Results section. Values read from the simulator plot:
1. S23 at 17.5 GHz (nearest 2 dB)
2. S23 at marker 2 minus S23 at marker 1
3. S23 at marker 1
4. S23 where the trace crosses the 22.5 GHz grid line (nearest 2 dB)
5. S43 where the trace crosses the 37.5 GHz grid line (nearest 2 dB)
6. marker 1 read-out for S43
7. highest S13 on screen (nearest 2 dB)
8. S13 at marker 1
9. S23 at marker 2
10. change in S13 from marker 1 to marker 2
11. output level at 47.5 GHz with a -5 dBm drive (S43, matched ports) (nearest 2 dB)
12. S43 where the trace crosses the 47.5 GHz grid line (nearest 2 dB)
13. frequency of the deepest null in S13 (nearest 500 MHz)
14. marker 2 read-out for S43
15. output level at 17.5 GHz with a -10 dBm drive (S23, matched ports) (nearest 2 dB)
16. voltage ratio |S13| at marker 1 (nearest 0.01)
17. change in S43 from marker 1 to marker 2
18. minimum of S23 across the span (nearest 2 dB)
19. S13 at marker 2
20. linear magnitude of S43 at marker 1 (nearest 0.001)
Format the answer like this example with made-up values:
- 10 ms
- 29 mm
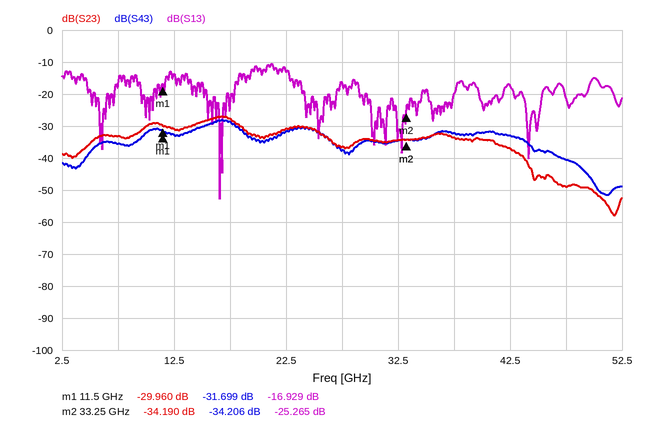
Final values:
- -28 dB
- -4.230 dB
- -29.960 dB
- -30 dB
- -32 dB
- -31.699 dB
- -10 dB
- -16.929 dB
- -34.190 dB
- -8.336 dB
- -46 dBm
- -40 dB
- 16.5 GHz
- -34.206 dB
- -38 dBm
- 0.14
- -2.507 dB
- -58 dB
- -25.265 dB
- 0.026
